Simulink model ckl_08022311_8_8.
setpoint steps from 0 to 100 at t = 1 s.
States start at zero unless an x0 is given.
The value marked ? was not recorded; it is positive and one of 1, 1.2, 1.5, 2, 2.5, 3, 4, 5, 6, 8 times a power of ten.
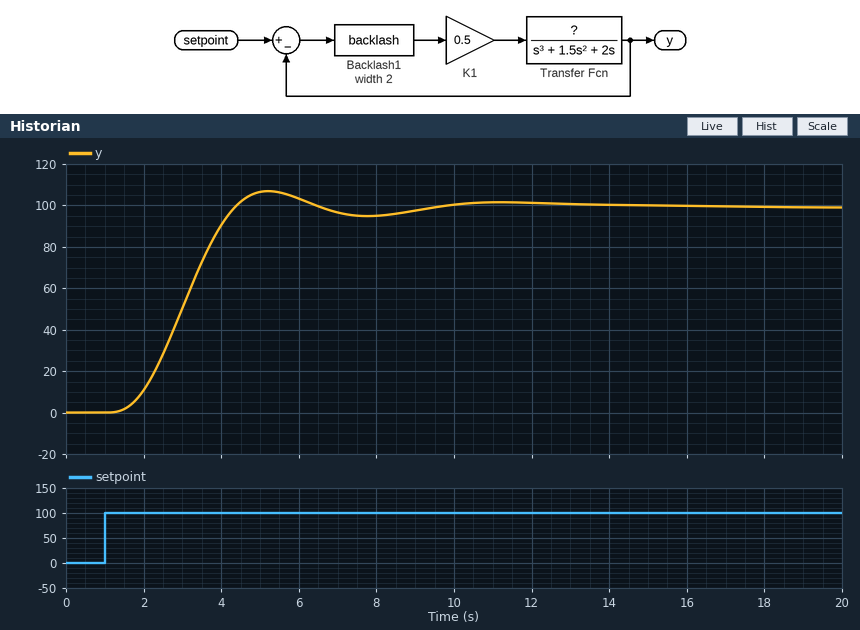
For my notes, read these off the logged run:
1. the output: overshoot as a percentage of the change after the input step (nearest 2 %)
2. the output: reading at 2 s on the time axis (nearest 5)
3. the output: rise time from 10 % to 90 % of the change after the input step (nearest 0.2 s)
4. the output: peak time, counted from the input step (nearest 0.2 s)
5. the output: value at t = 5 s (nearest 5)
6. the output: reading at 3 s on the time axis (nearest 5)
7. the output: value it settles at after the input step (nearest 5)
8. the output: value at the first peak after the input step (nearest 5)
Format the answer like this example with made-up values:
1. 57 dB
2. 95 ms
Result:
1. 8 %
2. 10
3. 2.0 s
4. 4.2 s
5. 105
6. 50
7. 100
8. 105
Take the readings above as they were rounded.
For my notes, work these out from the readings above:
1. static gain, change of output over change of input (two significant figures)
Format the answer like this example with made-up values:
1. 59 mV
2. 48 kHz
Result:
1. 1.0
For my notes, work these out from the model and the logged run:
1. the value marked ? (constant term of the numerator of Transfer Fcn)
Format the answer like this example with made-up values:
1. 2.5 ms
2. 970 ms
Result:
1. 2
